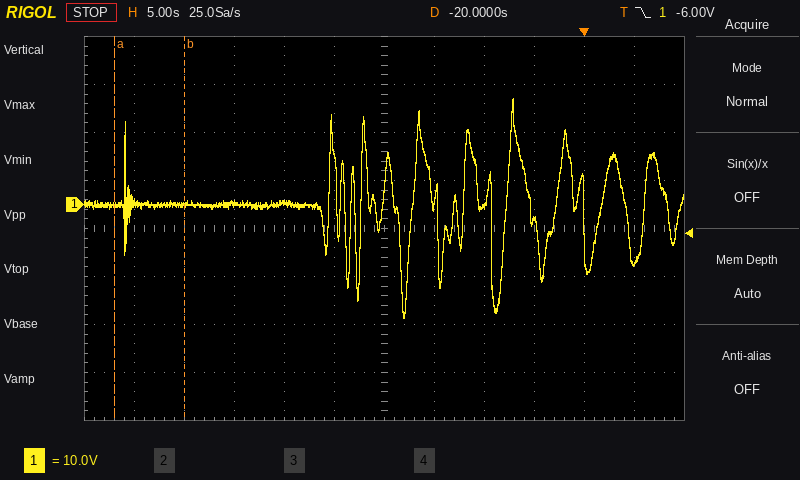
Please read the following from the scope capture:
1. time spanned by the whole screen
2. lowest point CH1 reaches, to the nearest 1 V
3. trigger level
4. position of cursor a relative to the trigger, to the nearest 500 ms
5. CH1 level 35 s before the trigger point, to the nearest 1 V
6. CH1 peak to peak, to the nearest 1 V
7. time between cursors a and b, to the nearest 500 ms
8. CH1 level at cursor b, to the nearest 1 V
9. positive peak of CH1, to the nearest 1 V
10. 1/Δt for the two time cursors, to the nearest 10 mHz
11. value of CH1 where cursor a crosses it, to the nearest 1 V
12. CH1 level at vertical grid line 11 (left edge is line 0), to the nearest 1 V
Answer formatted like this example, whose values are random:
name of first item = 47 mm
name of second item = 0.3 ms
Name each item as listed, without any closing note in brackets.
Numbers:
time spanned by the whole screen = 60 s
lowest point CH1 reaches, to the nearest 1 V = -24 V
trigger level = -6.00 V
position of cursor a relative to the trigger, to the nearest 500 ms = -47.0 s
CH1 level 35 s before the trigger point, to the nearest 1 V = 0 V
CH1 peak to peak, to the nearest 1 V = 46 V
time between cursors a and b, to the nearest 500 ms = 7.0 s
CH1 level at cursor b, to the nearest 1 V = 0 V
positive peak of CH1, to the nearest 1 V = 22 V
1/Δt for the two time cursors, to the nearest 10 mHz = 140 mHz
value of CH1 where cursor a crosses it, to the nearest 1 V = 0 V
CH1 level at vertical grid line 11 (left edge is line 0), to the nearest 1 V = -12 V
